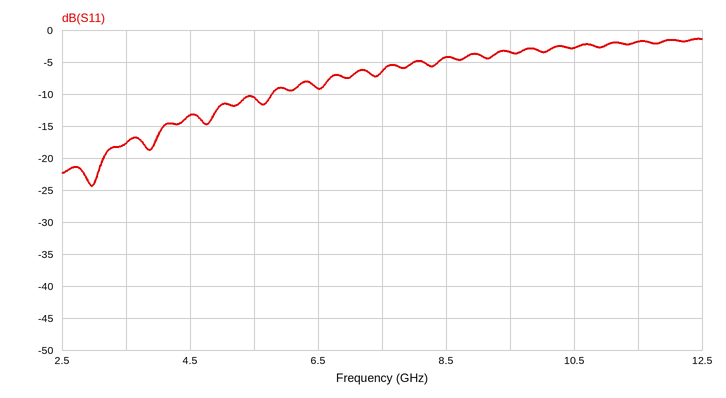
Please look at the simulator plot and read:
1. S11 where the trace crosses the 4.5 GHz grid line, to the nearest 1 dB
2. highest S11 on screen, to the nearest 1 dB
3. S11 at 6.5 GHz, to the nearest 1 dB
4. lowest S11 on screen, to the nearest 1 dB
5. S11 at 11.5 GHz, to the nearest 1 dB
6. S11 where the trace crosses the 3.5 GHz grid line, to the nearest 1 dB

-13 dB
-1 dB
-9 dB
-24 dB
-2 dB
-18 dB
